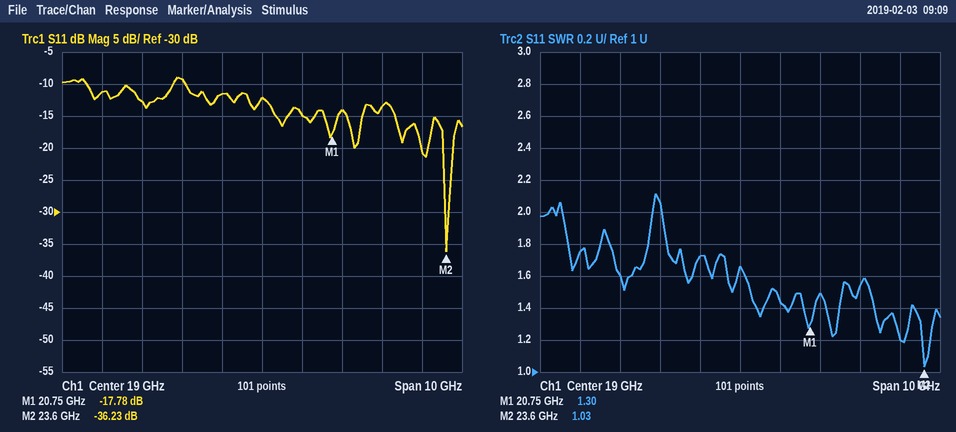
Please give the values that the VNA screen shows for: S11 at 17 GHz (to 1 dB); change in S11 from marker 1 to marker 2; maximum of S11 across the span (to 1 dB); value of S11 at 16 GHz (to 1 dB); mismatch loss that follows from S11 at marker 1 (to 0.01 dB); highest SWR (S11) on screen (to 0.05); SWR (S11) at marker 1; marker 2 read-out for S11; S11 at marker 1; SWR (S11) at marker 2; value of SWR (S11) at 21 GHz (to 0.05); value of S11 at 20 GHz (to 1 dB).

-9 dB
-18.45 dB
-9 dB
-13 dB
0.07 dB
2.10
1.30
-36.23 dB
-17.78 dB
1.03
1.50
-15 dB
